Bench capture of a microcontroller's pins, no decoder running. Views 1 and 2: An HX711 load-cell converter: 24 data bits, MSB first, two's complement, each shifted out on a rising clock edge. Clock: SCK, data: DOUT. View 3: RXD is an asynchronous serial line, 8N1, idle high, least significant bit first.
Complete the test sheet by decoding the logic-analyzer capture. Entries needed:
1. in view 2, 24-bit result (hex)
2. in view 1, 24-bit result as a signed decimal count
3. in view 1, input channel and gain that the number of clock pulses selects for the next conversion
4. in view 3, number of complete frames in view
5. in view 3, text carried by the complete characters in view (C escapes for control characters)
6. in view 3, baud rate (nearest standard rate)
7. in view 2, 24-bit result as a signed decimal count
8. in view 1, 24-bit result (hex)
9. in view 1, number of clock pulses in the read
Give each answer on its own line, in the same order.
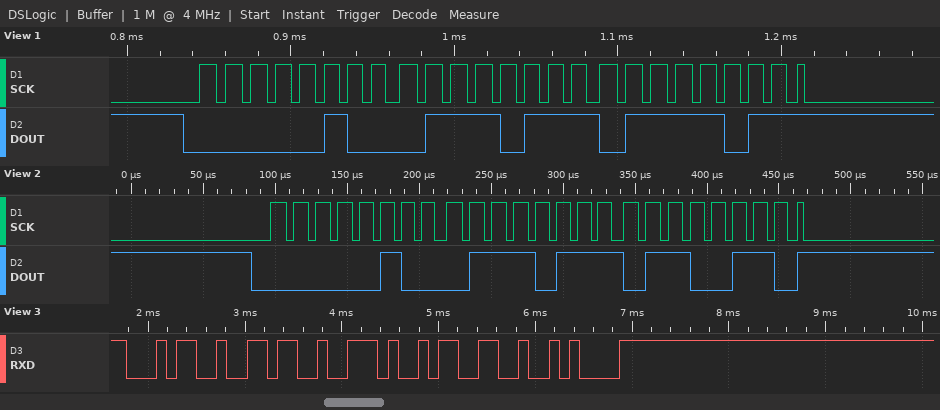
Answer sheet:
0x047766
292731
channel A, gain 128
5
"46.3\n"
9600 baud
292710
0x04777B
25
